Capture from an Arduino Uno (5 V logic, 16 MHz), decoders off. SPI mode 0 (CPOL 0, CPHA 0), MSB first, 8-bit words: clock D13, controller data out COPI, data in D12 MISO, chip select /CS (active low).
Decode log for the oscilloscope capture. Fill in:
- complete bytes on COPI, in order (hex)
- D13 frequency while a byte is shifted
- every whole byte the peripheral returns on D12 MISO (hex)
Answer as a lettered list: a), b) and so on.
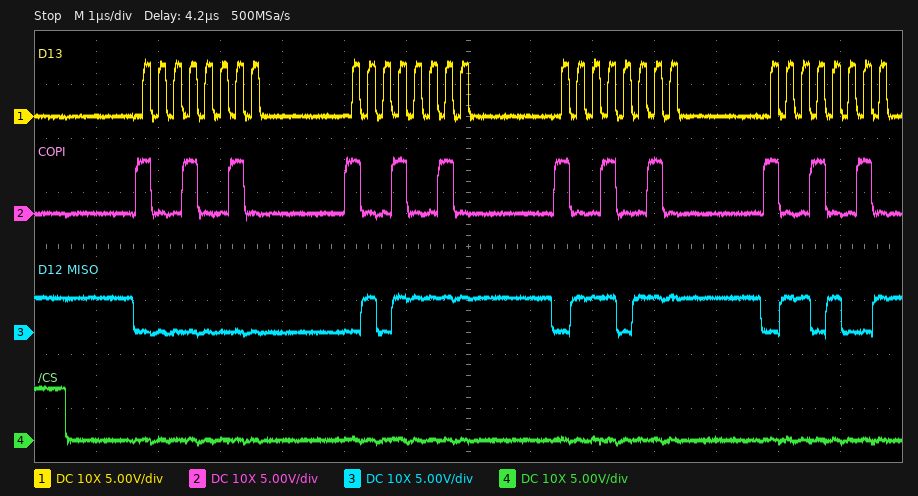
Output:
a) 92 92 92 92
b) 4 MHz
c) 00 5F 77 69
